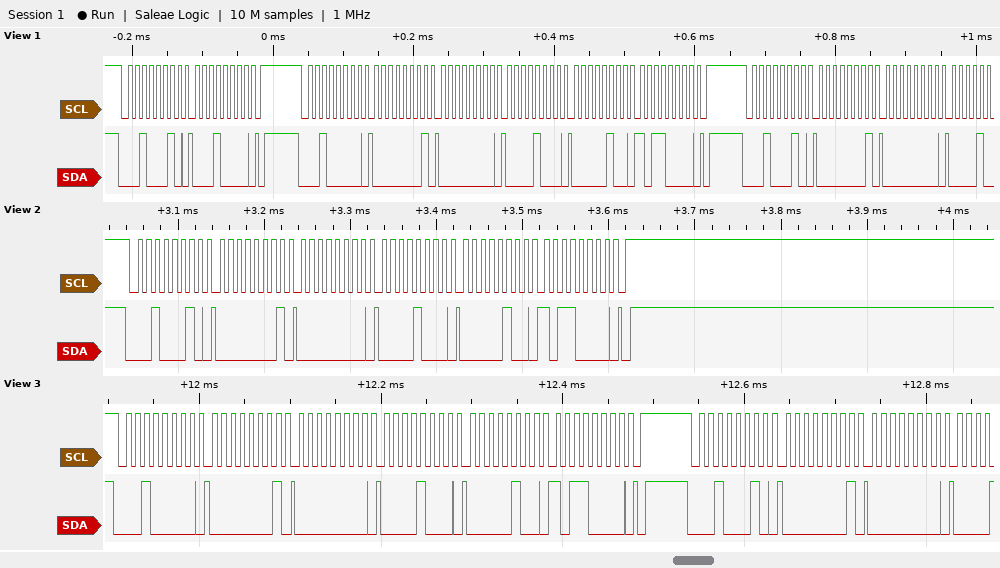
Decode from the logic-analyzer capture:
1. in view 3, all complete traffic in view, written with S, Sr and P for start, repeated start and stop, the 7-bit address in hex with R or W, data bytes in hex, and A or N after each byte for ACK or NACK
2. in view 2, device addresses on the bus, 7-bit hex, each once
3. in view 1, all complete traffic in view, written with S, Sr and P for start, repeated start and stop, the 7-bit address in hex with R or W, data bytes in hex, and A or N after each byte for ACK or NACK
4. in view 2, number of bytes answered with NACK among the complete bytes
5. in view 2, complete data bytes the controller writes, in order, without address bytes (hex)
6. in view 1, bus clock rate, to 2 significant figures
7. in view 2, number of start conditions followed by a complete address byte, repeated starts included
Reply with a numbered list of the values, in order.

1. S 10W A 01 A 00 A 08 A 04 A B0 A P S 11W A 01 A 00 A
2. 0x11
3. S 11W A 10 A P S 10W A 01 A 00 A 08 A 04 A B0 A P S 11W A 01 A 00 A
4. 0
5. 01 00 08 04 B0
6. 100 kHz
7. 1
